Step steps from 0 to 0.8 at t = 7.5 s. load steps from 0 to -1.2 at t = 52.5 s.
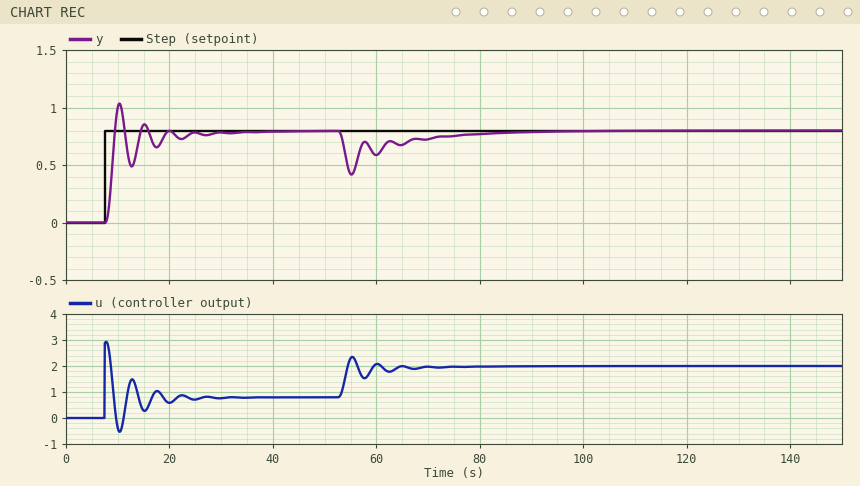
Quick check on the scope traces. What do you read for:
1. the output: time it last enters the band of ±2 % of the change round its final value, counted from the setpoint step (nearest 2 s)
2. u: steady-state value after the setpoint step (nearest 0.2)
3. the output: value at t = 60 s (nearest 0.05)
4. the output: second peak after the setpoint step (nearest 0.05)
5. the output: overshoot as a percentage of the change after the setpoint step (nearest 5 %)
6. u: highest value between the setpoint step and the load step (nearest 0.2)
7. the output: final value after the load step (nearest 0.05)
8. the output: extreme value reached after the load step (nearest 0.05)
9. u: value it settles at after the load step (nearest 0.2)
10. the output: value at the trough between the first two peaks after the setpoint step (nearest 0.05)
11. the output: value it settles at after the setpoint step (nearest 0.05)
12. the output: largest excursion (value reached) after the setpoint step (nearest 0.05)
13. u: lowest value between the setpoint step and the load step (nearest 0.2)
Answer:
26 s
0.8
0.60
0.85
30 %
3.0
0.80
0.40
2.0
0.50
0.80
1.05
-0.6
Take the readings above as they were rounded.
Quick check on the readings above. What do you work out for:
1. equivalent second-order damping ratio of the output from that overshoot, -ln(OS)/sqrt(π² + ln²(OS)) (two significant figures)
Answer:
0.36
